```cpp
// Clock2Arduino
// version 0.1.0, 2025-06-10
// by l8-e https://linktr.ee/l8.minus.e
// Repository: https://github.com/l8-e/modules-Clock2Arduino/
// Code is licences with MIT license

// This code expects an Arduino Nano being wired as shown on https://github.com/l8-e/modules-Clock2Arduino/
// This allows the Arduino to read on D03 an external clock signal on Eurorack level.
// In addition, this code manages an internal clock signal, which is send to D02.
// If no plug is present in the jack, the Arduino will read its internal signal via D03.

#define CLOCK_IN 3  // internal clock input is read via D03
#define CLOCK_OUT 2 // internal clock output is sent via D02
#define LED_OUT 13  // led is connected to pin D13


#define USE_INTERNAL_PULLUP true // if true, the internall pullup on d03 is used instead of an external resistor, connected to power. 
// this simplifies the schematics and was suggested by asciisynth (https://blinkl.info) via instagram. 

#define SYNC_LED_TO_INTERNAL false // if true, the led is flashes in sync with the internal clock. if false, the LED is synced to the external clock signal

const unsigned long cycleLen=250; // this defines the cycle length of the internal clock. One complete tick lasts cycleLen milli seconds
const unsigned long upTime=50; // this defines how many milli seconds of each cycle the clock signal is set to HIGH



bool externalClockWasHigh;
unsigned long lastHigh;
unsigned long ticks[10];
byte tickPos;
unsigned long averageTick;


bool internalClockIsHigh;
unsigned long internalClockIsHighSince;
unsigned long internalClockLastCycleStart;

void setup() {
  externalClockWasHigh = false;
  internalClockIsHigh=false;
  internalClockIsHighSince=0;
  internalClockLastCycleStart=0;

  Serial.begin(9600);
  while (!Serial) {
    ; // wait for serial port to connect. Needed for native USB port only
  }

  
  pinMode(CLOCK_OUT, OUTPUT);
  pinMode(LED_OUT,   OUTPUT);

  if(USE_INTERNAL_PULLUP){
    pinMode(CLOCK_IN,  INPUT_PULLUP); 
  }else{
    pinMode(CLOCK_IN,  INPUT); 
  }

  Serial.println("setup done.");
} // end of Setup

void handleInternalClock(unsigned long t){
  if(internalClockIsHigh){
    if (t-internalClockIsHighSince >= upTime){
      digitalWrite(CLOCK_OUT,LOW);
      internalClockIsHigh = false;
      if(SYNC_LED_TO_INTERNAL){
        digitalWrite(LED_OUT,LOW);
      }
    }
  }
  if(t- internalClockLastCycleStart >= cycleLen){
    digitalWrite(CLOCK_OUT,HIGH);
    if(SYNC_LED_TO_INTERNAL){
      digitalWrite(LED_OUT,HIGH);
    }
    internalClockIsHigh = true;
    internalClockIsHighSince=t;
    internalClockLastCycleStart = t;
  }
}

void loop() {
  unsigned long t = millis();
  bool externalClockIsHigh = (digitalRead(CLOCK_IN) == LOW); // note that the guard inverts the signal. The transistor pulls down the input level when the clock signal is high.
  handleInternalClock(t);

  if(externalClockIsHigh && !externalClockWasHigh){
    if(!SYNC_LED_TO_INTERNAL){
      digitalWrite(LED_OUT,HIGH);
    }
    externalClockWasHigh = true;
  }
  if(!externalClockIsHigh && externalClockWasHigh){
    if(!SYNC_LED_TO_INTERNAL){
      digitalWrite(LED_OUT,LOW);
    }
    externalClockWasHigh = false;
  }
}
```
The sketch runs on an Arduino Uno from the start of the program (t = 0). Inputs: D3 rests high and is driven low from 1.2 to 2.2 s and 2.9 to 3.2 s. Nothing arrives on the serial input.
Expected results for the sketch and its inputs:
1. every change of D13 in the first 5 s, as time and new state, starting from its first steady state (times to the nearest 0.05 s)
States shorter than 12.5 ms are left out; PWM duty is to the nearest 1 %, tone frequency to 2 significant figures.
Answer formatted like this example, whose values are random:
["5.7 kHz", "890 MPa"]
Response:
["0 s low; 1.2 s high; 2.2 s low; 2.9 s high; 3.2 s low"]
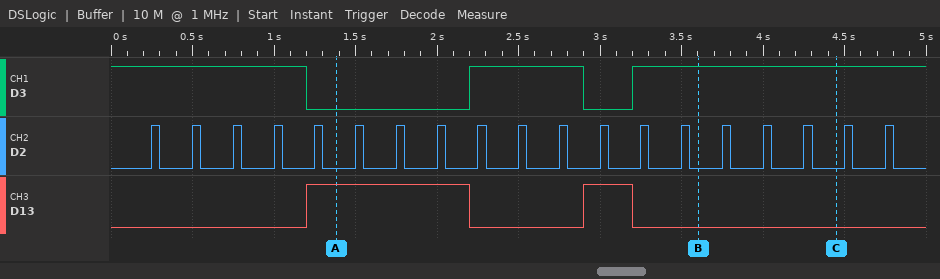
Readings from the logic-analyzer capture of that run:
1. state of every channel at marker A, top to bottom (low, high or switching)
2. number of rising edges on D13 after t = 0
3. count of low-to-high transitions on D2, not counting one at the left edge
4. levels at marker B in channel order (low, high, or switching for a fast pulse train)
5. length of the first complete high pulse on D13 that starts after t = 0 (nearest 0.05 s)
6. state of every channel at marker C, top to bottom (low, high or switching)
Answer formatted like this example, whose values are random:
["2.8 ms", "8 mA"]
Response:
["D3 low, D2 low, D13 high", "2", "19", "D3 high, D2 low, D13 low", "1.00 s", "D3 high, D2 low, D13 low"]
